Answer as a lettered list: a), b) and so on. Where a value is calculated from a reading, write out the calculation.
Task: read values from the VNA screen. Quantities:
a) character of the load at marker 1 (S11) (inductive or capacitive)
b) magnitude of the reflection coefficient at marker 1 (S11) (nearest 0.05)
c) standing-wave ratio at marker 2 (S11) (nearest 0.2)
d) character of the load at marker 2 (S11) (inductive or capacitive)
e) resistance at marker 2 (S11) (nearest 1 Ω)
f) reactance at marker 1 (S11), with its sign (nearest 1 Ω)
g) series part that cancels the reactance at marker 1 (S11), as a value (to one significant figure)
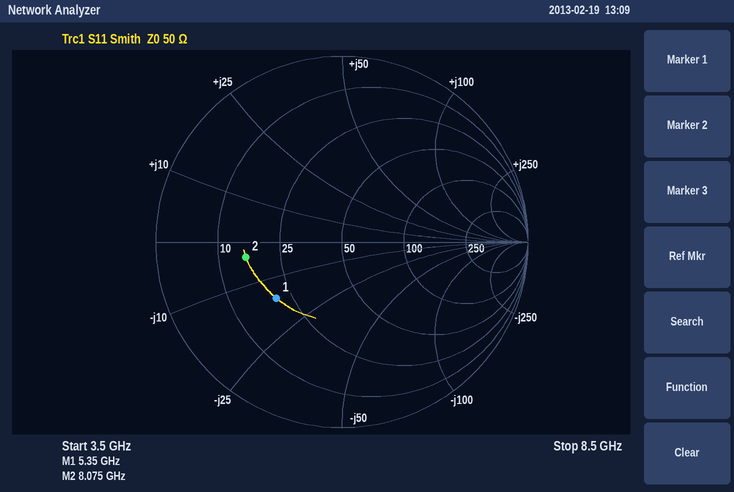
a) capacitive
b) 0.45
c) 3.2
d) capacitive
e) 16 Ω
f) -16 Ω
g) L = 16 Ω/(2π × 5.35 GHz) ≈ 476 pH, so 500 pH to one significant figure
